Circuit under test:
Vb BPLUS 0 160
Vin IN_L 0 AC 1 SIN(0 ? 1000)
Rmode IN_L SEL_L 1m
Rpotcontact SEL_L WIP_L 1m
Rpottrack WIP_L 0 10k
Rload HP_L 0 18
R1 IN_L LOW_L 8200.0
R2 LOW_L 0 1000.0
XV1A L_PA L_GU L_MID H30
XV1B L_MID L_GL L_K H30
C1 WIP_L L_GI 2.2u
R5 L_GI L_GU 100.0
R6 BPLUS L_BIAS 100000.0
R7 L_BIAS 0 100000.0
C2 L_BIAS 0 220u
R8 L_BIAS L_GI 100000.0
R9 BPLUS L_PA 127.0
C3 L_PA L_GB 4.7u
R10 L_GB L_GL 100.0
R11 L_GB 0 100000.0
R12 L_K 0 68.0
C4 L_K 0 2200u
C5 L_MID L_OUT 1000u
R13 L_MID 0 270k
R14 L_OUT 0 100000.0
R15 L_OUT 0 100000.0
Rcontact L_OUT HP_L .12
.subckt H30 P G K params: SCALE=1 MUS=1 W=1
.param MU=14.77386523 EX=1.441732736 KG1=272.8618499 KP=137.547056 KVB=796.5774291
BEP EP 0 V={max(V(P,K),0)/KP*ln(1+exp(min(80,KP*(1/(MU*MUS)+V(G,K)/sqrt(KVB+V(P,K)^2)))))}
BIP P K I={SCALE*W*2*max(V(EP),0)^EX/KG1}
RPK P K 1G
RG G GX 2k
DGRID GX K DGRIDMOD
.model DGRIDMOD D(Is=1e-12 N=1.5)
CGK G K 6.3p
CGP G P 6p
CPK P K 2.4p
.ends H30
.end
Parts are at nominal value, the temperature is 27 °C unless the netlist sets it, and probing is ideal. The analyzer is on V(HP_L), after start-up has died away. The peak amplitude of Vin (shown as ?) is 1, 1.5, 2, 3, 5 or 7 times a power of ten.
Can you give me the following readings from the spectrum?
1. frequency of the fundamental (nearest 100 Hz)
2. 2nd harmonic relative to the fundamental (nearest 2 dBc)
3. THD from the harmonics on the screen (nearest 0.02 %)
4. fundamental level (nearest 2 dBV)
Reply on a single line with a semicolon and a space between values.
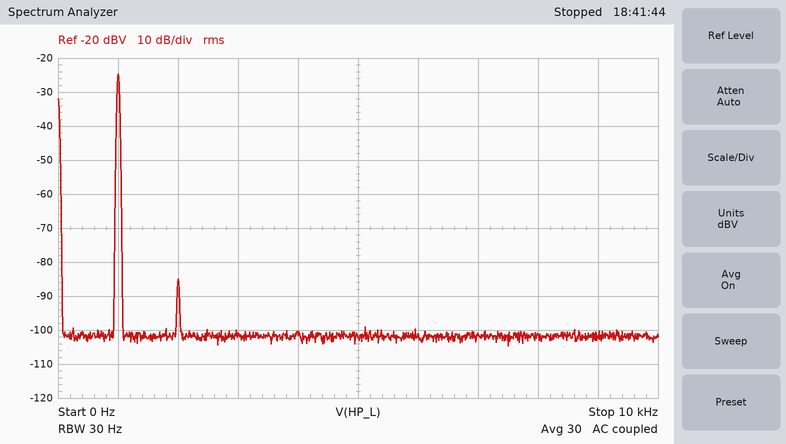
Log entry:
1.0 kHz; -60 dBc; 0.10 %; -24 dBV
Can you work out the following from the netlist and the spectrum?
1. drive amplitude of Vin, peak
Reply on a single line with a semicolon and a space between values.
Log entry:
200 mV
